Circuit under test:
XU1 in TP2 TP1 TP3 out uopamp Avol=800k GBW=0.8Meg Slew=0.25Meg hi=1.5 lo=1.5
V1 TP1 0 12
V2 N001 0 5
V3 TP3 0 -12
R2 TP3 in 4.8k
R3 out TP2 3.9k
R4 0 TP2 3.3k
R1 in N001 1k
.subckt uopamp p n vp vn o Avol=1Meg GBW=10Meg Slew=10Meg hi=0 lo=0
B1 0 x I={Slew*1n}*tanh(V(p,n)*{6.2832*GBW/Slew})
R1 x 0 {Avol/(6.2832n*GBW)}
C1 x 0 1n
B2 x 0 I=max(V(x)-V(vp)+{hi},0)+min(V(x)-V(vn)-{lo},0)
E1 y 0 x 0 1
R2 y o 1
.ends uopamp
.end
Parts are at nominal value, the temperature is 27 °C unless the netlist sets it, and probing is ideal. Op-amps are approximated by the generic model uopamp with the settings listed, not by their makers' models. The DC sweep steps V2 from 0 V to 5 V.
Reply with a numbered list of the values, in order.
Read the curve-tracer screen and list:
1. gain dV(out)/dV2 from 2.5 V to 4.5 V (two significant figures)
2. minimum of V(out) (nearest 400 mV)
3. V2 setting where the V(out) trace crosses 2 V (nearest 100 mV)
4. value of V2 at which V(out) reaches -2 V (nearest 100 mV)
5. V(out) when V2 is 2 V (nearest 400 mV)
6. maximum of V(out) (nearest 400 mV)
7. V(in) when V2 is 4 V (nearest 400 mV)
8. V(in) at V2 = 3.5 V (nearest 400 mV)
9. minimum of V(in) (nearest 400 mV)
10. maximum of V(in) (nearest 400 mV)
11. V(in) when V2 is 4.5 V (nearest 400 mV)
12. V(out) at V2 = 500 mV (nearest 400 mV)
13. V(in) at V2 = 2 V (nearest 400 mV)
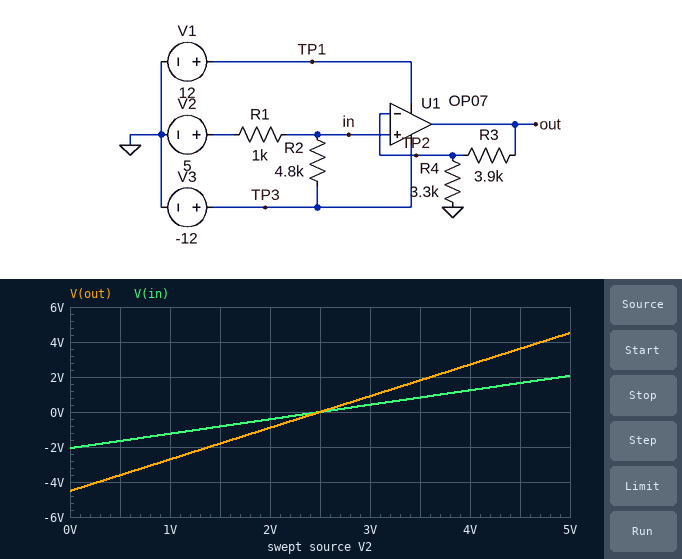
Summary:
1. 1.8 V/V
2. -4.4 V
3. 3.6 V
4. 1.4 V
5. -800 mV
6. 4.4 V
7. 1.2 V
8. 800 mV
9. -2.0 V
10. 2.0 V
11. 1.6 V
12. -3.6 V
13. -400 mV
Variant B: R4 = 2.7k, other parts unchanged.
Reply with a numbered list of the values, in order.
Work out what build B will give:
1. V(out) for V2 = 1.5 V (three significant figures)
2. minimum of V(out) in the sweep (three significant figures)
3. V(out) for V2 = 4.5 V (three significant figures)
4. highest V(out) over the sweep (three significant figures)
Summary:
1. -2.02 V
2. -5.06 V
3. 4.05 V
4. 5.06 V
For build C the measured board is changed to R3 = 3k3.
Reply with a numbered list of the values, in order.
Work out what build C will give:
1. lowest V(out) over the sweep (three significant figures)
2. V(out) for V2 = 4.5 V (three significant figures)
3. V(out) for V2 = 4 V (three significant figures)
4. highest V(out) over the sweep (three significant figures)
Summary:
1. -4.14 V
2. 3.31 V
3. 2.48 V
4. 4.14 V
